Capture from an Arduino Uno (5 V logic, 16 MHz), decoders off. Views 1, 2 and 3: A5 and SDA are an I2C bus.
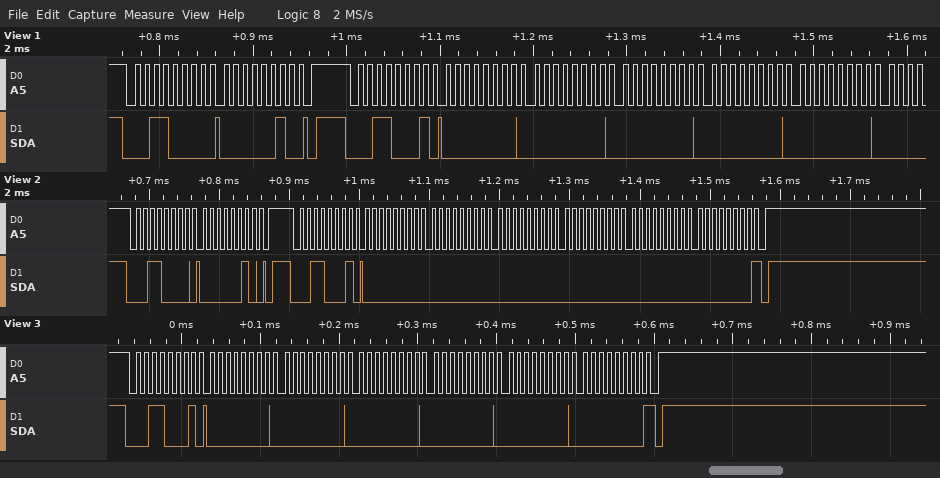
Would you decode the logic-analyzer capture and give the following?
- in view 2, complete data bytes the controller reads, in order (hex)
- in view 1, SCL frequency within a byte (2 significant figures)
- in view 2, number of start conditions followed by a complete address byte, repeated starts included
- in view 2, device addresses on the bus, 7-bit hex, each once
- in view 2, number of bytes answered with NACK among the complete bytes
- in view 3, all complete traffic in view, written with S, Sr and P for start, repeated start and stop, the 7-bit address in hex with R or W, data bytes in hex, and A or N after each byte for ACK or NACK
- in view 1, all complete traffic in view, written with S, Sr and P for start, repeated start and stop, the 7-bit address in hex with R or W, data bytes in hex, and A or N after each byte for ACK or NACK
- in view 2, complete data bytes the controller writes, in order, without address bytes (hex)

00 00 00 00 00 00
100 kHz
2
0x18
1
S 18R A 00 A 00 A 00 A 00 A 00 A 00 N P
S 18W A 02 A P S 18R A 00 A 00 A 00 A 00 A 00 A
02
